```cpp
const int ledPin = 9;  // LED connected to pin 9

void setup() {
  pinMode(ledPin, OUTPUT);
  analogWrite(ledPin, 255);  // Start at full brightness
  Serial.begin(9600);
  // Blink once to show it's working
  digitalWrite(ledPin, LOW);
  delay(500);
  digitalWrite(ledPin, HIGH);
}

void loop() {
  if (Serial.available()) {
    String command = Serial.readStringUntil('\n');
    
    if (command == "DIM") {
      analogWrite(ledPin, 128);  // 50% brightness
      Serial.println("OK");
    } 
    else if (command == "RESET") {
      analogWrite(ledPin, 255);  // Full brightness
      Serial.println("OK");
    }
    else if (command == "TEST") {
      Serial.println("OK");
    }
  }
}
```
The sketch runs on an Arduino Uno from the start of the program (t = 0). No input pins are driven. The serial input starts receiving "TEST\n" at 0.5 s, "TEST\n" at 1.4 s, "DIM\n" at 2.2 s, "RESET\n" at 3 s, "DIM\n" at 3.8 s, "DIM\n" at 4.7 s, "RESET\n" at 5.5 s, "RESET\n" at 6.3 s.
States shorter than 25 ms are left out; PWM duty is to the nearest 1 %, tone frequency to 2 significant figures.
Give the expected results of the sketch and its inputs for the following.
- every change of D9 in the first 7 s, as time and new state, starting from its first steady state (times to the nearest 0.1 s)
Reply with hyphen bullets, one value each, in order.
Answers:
- 0 s low; 0.5 s high; 2.2 s PWM 50 %; 3 s high; 3.8 s PWM 50 %; 5.5 s high
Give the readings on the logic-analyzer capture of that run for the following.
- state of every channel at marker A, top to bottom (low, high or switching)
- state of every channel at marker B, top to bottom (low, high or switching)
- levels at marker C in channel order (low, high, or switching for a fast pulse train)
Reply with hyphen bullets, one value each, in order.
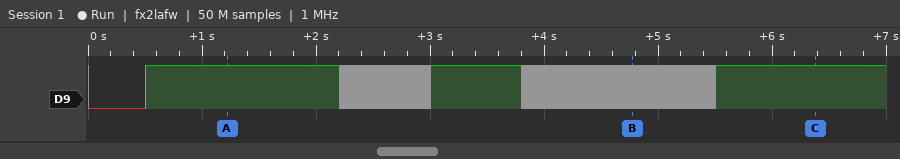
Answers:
- D9 high
- D9 switching
- D9 high
